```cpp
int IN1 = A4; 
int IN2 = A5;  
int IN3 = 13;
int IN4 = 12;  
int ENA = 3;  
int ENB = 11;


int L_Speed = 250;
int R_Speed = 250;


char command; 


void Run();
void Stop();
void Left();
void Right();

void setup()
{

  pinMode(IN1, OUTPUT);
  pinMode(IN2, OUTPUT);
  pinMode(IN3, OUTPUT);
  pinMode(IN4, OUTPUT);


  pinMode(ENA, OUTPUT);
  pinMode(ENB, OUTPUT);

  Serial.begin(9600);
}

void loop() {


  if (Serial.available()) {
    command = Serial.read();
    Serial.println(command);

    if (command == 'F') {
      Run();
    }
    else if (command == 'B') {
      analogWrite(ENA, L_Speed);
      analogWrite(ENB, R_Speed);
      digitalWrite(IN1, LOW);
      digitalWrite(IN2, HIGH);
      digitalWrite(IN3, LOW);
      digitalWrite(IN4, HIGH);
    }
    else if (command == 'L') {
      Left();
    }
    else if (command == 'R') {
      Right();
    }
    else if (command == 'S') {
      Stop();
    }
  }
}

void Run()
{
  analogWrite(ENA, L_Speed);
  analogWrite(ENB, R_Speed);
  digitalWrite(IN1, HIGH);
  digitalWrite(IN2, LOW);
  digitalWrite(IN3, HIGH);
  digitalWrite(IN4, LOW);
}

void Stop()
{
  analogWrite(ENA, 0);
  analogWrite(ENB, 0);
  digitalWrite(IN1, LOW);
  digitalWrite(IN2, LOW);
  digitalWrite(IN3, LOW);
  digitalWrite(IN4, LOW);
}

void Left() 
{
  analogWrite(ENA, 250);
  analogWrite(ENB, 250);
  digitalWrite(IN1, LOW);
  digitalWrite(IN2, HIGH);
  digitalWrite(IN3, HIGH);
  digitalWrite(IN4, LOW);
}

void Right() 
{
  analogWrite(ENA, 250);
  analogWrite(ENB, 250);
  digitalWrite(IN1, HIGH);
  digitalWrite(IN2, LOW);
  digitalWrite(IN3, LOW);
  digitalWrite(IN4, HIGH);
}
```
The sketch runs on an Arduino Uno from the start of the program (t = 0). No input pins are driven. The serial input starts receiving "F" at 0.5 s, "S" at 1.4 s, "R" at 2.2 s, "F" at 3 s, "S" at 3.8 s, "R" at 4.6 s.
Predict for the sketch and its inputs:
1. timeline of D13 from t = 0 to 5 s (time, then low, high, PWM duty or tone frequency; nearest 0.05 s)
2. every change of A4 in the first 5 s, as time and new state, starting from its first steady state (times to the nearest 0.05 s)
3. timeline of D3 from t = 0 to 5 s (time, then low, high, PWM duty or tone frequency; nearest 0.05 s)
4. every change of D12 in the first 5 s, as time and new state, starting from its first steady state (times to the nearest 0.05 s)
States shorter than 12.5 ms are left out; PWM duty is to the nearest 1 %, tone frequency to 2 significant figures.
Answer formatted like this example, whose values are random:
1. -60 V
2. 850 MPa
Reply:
1. 0 s low; 0.5 s high; 1.4 s low; 3 s high; 3.8 s low
2. 0 s low; 0.5 s high; 1.4 s low; 2.2 s high; 3.8 s low; 4.6 s high
3. 0 s low; 0.5 s PWM 98 %; 1.4 s low; 2.2 s PWM 98 %; 3.8 s low; 4.6 s PWM 98 %
4. 0 s low; 2.2 s high; 3 s low; 4.6 s high
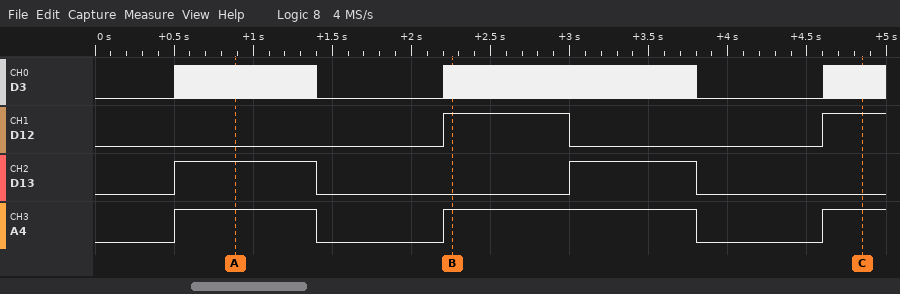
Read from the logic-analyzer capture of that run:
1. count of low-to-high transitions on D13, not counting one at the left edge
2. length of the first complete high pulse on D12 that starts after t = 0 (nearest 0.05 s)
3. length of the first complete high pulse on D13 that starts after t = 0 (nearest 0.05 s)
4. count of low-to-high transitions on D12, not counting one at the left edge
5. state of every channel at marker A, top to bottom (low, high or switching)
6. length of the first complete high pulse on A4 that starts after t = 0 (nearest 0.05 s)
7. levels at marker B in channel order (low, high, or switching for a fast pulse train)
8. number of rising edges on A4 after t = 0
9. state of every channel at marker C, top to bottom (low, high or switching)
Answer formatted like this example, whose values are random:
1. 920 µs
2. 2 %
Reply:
1. 2
2. 0.80 s
3. 0.90 s
4. 2
5. D3 switching, D12 low, D13 high, A4 high
6. 0.90 s
7. D3 switching, D12 high, D13 low, A4 high
8. 3
9. D3 switching, D12 high, D13 low, A4 high
